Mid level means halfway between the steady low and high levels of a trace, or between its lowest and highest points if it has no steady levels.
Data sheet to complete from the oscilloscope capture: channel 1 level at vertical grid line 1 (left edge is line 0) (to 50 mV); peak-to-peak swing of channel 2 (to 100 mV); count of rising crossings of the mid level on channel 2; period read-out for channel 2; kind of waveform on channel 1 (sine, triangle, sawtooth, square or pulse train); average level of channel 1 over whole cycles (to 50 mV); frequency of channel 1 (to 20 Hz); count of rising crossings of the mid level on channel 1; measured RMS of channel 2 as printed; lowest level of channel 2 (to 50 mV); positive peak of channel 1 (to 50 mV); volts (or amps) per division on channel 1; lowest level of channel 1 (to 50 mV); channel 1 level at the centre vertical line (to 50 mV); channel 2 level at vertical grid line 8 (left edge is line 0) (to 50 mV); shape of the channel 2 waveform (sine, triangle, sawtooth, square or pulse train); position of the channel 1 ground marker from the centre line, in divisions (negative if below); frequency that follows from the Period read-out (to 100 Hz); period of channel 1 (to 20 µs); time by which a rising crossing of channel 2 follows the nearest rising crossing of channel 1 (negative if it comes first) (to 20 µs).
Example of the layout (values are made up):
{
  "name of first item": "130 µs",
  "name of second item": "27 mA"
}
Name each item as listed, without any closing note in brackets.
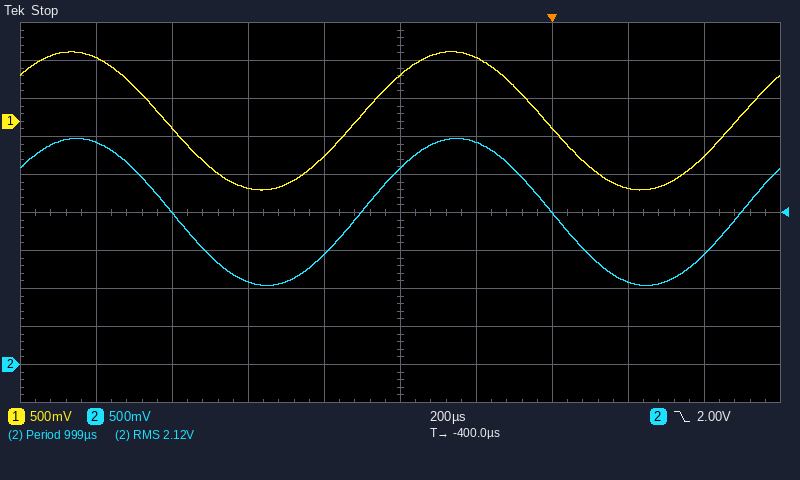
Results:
{
  "channel 1 level at vertical grid line 1 (left edge is line 0)": "850 mV",
  "peak-to-peak swing of channel 2": "1.90 V",
  "count of rising crossings of the mid level on channel 2": "2",
  "period read-out for channel 2": "999 µs",
  "kind of waveform on channel 1": "sine",
  "average level of channel 1 over whole cycles": "0 mV",
  "frequency of channel 1": "1.00 kHz",
  "count of rising crossings of the mid level on channel 1": "2",
  "measured RMS of channel 2 as printed": "2.12 V",
  "lowest level of channel 2": "1.05 V",
  "positive peak of channel 1": "900 mV",
  "volts (or amps) per division on channel 1": "500 mV",
  "lowest level of channel 1": "-900 mV",
  "channel 1 level at the centre vertical line": "600 mV",
  "channel 2 level at vertical grid line 8 (left edge is line 0)": "1.10 V",
  "shape of the channel 2 waveform": "sine",
  "position of the channel 1 ground marker from the centre line, in divisions": "+2.4 div",
  "frequency that follows from the Period read-out": "1.0 kHz",
  "period of channel 1": "1.00 ms",
  "time by which a rising crossing of channel 2 follows the nearest rising crossing of channel 1 (negative if it comes first)": "+20 µs"
}
